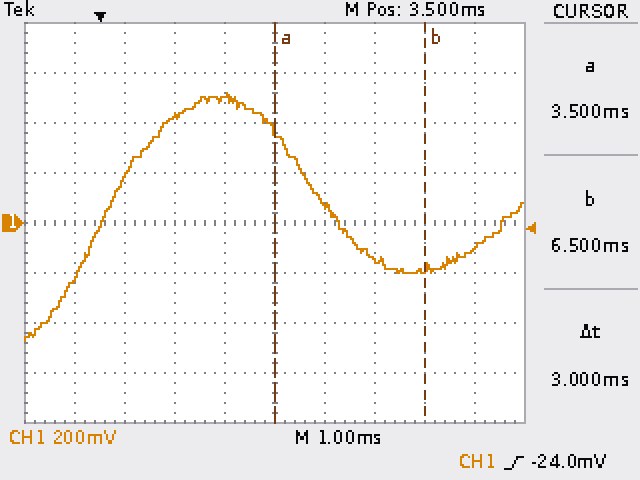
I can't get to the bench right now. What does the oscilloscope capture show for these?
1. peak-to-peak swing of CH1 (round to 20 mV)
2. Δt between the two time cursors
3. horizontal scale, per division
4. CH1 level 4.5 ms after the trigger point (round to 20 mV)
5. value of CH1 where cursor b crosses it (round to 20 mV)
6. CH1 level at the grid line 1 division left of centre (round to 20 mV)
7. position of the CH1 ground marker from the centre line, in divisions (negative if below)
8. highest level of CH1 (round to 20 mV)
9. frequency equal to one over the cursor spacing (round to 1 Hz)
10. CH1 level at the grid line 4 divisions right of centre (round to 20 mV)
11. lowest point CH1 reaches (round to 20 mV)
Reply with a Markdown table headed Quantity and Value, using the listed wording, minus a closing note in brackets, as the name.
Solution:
| Quantity | Value |
|---|---|
| peak-to-peak swing of CH1 | 1.00 V |
| Δt between the two time cursors | 3 ms |
| horizontal scale, per division | 1 ms |
| CH1 level 4.5 ms after the trigger point | 80 mV |
| value of CH1 where cursor b crosses it | -180 mV |
| CH1 level at the grid line 1 division left of centre | 500 mV |
| position of the CH1 ground marker from the centre line, in divisions | 0.0 div |
| highest level of CH1 | 520 mV |
| frequency equal to one over the cursor spacing | 333 Hz |
| CH1 level at the grid line 4 divisions right of centre | -100 mV |
| lowest point CH1 reaches | -480 mV |
